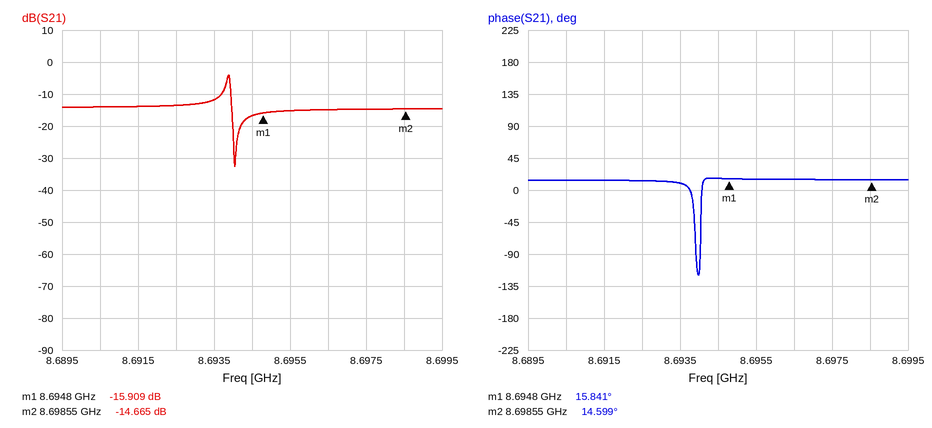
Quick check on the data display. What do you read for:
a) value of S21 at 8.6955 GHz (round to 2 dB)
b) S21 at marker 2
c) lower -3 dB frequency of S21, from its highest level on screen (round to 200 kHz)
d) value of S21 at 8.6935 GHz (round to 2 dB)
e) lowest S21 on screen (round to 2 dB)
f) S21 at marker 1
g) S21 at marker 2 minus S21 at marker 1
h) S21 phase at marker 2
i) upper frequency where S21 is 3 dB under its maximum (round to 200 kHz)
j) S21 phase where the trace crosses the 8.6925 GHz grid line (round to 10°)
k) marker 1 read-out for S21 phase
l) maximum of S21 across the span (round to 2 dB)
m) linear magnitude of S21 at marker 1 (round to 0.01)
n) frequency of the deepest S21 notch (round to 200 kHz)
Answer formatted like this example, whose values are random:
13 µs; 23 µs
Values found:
-16 dB; -14.665 dB; 8.6938 GHz; -12 dB; -32 dB; -15.909 dB; 1.244 dB; 14.599°; 8.6940 GHz; 10°; 15.841°; -4 dB; 0.16; 8.6940 GHz
